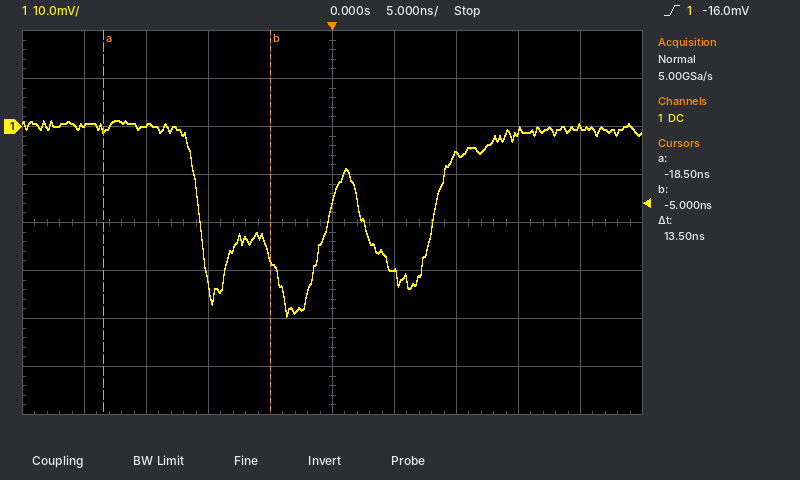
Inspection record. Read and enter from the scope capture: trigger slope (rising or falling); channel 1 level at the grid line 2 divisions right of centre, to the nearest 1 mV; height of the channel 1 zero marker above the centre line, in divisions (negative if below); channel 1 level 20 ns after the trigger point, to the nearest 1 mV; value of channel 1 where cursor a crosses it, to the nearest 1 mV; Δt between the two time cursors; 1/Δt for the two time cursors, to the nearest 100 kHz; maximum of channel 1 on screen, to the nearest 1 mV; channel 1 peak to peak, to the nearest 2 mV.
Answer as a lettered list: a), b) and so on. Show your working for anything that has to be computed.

a) rising
b) -6 mV
c) +2.0 div
d) 0 mV
e) 0 mV
f) 13.5 ns
g) 1 / 13.5 ns ≈ 74.1 MHz
h) 1 mV
i) 40 mV
